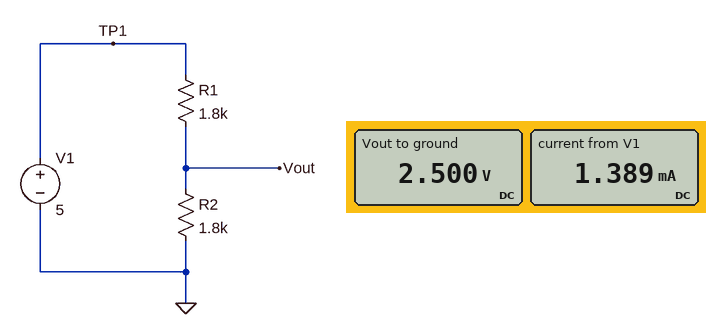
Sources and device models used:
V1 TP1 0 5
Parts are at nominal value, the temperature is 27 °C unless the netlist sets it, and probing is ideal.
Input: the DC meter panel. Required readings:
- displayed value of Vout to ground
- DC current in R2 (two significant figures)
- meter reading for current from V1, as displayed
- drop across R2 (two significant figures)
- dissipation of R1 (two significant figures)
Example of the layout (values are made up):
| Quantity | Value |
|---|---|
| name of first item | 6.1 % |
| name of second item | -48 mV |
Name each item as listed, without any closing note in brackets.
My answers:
| Quantity | Value |
|---|---|
| displayed value of Vout to ground | 2.500 V |
| DC current in R2 | 1.4 mA |
| meter reading for current from V1, as displayed | 1.389 mA |
| drop across R2 | 2.5 V |
| dissipation of R1 | 3.5 mW |
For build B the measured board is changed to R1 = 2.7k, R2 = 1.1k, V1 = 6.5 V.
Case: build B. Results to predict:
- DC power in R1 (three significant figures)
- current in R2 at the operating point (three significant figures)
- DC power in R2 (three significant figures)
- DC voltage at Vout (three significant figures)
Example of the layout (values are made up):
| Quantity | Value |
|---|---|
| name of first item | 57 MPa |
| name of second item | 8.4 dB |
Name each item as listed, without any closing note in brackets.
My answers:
| Quantity | Value |
|---|---|
| DC power in R1 | 7.90 mW |
| current in R2 at the operating point | 1.71 mA |
| DC power in R2 | 3.22 mW |
| DC voltage at Vout | 1.88 V |
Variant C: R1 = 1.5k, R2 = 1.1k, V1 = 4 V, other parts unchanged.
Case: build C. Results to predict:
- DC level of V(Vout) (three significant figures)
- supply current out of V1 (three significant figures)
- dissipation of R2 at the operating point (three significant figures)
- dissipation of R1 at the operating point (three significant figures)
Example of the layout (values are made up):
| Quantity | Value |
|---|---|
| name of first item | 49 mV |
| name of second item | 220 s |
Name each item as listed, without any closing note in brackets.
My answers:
| Quantity | Value |
|---|---|
| DC level of V(Vout) | 1.69 V |
| supply current out of V1 | 1.54 mA |
| dissipation of R2 at the operating point | 2.60 mW |
| dissipation of R1 at the operating point | 3.55 mW |
